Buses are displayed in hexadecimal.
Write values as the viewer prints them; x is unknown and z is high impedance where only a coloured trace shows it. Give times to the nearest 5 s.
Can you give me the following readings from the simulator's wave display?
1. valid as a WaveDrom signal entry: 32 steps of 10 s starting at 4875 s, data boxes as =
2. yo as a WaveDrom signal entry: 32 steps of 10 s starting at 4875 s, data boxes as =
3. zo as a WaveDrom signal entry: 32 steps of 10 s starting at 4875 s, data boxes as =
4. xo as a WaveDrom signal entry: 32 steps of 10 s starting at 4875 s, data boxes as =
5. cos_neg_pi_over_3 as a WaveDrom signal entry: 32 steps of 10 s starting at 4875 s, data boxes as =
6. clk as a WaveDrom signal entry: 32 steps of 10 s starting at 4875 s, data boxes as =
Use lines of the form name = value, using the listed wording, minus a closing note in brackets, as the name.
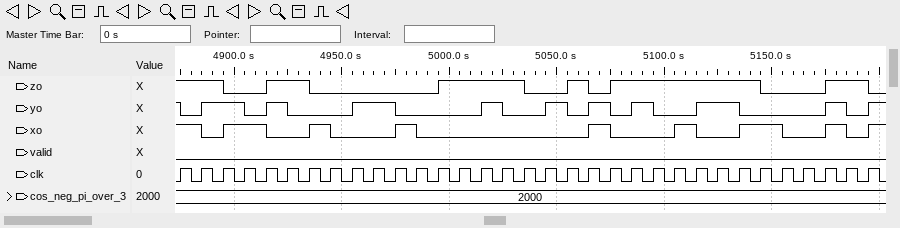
valid as a WaveDrom signal entry: 32 steps of 10 s starting at 4875 s, data boxes as = = {name: 'valid', wave: '0...............................'}
yo as a WaveDrom signal entry: 32 steps of 10 s starting at 4875 s, data boxes as = = {name: 'yo', wave: '01.010..1.0...10.101010.1.0...10'}
zo as a WaveDrom signal entry: 32 steps of 10 s starting at 4875 s, data boxes as = = {name: 'zo', wave: '1.0.1.0.....1...0.101......0..1.'}
xo as a WaveDrom signal entry: 32 steps of 10 s starting at 4875 s, data boxes as = = {name: 'xo', wave: '101.0.10..10.......10..10.1.0.10'}
cos_neg_pi_over_3 as a WaveDrom signal entry: 32 steps of 10 s starting at 4875 s, data boxes as = = {name: 'cos_neg_pi_over_3', wave: '=...............................', data: '2000'}
clk as a WaveDrom signal entry: 32 steps of 10 s starting at 4875 s, data boxes as = = {name: 'clk', wave: 'p...............................'}
